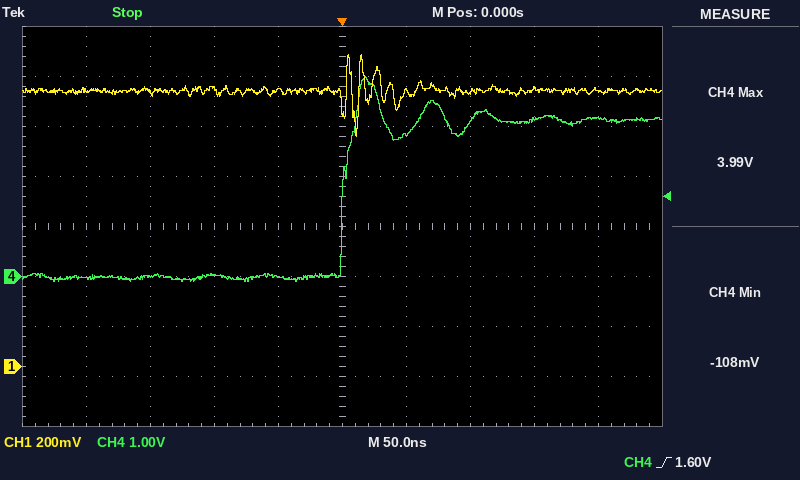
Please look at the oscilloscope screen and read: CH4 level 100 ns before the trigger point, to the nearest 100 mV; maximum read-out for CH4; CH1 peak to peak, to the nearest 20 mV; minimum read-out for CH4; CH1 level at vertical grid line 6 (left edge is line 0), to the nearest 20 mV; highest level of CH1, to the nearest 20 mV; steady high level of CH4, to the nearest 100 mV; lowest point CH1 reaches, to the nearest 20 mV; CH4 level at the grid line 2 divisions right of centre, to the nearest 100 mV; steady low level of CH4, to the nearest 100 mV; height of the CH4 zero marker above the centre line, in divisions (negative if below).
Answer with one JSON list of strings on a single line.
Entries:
["0.0 V", "3.99 V", "320 mV", "-108 mV", "1.10 V", "1.24 V", "3.1 V", "920 mV", "3.1 V", "0.0 V", "-1.0 div"]
